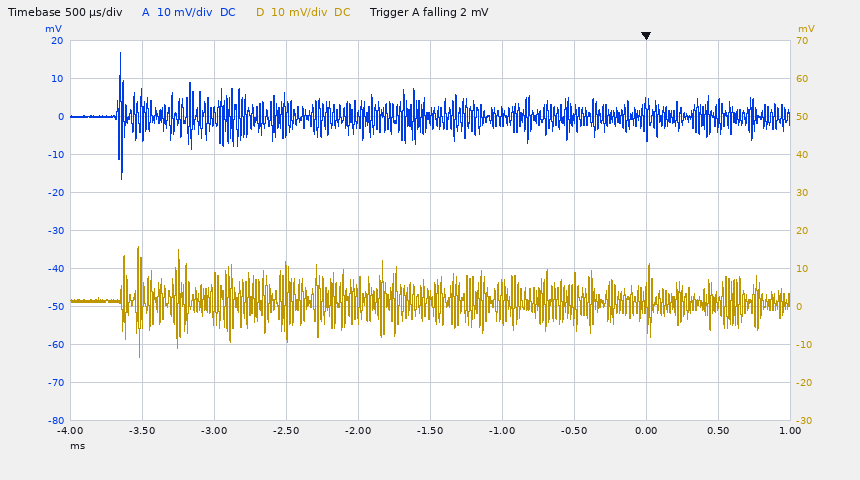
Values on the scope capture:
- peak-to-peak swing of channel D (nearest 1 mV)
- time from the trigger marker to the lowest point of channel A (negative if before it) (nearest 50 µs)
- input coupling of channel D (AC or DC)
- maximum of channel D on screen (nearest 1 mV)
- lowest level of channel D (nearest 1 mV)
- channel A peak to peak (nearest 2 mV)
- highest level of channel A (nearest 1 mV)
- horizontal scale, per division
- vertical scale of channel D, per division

29 mV
-3.65 ms
DC
16 mV
-13 mV
34 mV
17 mV
500 µs
10 mV
